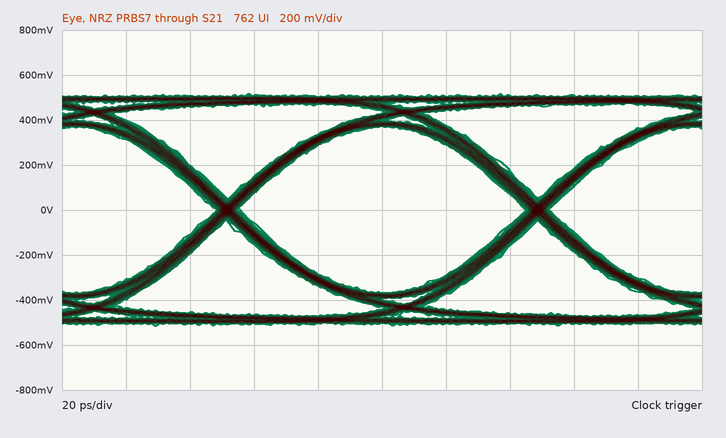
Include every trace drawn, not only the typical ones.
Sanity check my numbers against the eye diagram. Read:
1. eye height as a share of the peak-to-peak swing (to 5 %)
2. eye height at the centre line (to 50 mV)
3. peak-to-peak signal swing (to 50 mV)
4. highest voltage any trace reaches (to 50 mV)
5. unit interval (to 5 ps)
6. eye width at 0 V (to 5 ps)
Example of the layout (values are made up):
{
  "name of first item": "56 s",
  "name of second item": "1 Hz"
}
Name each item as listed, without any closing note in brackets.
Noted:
{
  "eye height as a share of the peak-to-peak swing": "70 %",
  "eye height at the centre line": "750 mV",
  "peak-to-peak signal swing": "1.05 V",
  "highest voltage any trace reaches": "500 mV",
  "unit interval": "95 ps",
  "eye width at 0 V": "90 ps"
}
